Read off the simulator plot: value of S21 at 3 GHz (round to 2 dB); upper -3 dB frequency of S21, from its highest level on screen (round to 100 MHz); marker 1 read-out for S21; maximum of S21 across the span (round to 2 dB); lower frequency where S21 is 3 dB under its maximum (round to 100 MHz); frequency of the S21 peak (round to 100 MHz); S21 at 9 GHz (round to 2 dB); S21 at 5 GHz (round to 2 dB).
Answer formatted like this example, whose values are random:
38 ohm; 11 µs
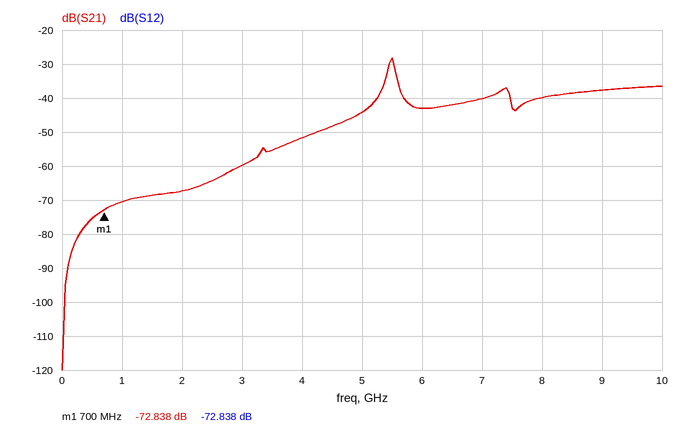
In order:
-60 dB; 5.5 GHz; -72.838 dB; -28 dB; 5.4 GHz; 5.5 GHz; -38 dB; -44 dB
